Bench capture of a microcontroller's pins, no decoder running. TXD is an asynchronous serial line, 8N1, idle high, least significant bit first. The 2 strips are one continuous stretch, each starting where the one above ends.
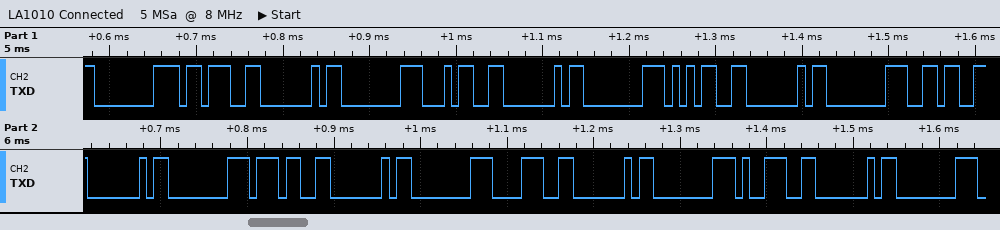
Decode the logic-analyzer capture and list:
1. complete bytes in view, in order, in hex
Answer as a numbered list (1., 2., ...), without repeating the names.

1. 80 3B 40 80 34 40 80 35 40 80 36 40 80 37 40 80 38 40 80 39 40 80
